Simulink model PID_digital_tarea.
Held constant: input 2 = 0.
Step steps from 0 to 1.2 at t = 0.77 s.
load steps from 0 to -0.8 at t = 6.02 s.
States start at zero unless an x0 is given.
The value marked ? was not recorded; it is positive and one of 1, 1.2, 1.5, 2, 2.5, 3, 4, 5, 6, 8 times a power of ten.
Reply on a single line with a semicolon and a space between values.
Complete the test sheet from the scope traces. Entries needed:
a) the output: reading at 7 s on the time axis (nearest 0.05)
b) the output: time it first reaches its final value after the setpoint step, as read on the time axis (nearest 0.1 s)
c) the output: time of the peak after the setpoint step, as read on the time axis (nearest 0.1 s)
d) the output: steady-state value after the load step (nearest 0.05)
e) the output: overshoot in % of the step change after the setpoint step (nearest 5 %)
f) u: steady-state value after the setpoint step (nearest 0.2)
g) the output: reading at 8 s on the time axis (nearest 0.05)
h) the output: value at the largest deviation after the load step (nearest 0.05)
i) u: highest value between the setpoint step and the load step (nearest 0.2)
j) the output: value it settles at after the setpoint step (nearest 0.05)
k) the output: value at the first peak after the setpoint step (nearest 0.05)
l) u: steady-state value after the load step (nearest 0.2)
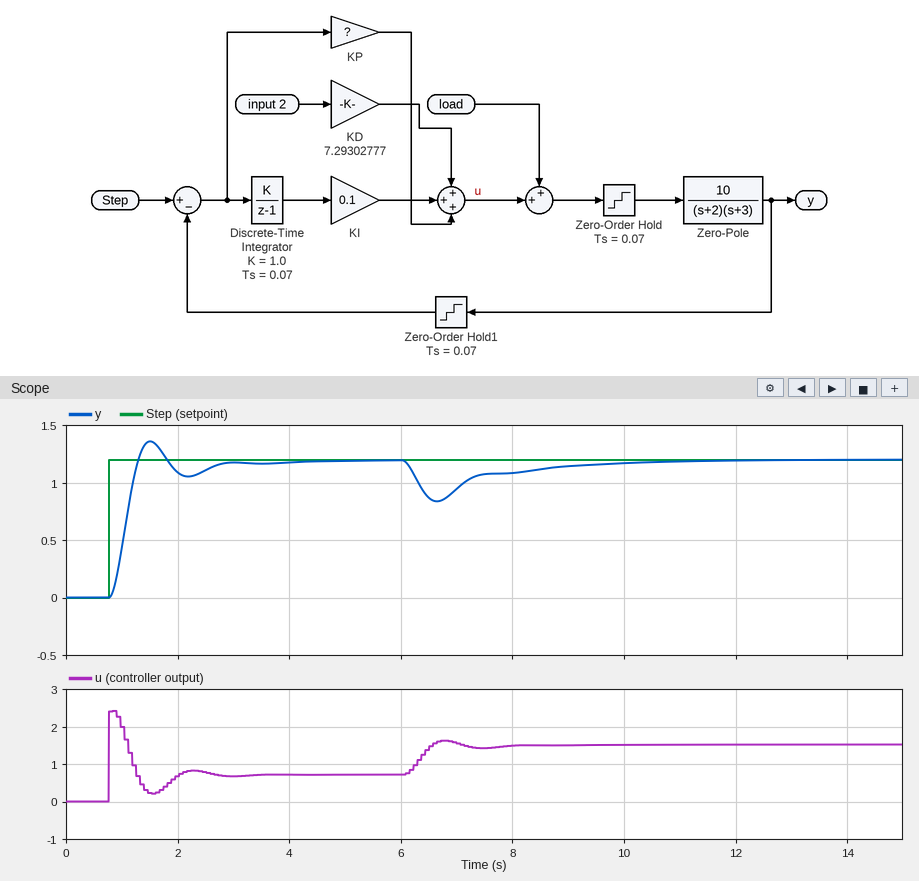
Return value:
0.95; 1.3 s; 1.5 s; 1.20; 15 %; 0.8; 1.10; 0.85; 2.4; 1.20; 1.35; 1.6
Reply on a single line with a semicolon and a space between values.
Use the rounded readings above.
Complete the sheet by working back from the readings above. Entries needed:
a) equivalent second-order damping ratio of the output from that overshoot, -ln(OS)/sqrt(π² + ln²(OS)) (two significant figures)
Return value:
0.52
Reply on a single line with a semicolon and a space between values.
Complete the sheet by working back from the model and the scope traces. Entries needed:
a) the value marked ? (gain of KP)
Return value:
2
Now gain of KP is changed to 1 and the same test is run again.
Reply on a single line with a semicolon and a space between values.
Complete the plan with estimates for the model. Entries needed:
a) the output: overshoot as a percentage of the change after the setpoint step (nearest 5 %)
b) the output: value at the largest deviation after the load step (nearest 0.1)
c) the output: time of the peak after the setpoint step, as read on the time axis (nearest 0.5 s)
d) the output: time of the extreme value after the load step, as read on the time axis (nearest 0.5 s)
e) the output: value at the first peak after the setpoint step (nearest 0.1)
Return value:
10 %; 0.7; 2.0 s; 7.0 s; 1.3
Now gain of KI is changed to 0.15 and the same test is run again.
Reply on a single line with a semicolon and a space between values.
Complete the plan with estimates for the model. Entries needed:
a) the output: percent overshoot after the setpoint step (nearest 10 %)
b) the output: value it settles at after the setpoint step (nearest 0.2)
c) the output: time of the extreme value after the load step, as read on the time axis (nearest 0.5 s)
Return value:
20 %; 1.2; 6.5 s
